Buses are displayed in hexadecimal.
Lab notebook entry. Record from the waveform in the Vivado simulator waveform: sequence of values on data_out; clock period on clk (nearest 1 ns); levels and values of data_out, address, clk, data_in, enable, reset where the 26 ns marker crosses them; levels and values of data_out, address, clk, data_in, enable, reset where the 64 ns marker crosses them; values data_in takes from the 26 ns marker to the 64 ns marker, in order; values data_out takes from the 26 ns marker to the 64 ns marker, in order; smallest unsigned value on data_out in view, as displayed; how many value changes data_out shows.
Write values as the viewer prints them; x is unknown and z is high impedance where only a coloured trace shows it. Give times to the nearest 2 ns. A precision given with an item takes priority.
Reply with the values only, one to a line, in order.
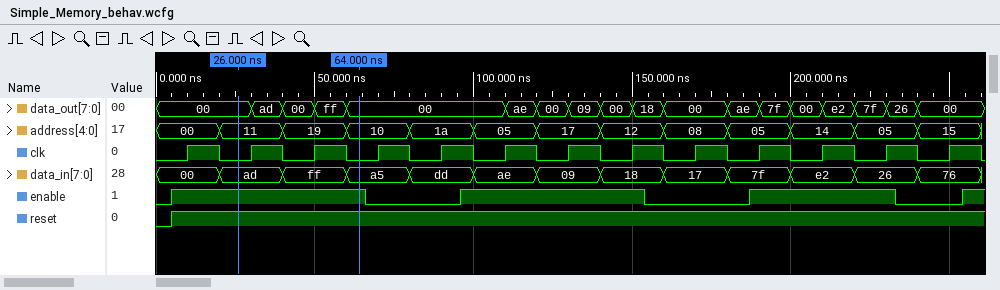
00, ad, 00, ff, 00, ae, 00, 09, 00, 18, 00, ae, 7f, 00, e2, 7f, 26, 00
20 ns
data_out=00, address=11, clk=0, data_in=ad, enable=1, reset=1
data_out=00, address=10, clk=0, data_in=a5, enable=1, reset=1
ad, ff, a5
00, ad, 00, ff, 00
00
17
